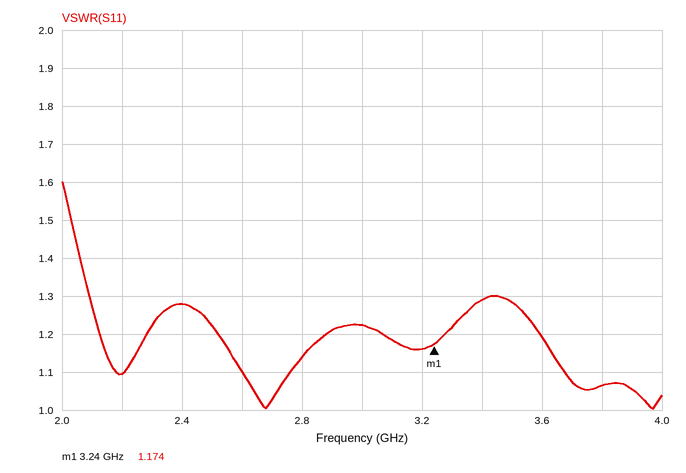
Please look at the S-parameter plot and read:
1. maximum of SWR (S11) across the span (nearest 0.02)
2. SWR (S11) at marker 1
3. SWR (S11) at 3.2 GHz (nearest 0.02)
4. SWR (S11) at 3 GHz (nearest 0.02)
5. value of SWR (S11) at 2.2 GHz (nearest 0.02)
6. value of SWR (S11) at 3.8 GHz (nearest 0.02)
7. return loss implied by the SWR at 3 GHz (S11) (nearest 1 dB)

1.60
1.174
1.16
1.22
1.10
1.06
20 dB
